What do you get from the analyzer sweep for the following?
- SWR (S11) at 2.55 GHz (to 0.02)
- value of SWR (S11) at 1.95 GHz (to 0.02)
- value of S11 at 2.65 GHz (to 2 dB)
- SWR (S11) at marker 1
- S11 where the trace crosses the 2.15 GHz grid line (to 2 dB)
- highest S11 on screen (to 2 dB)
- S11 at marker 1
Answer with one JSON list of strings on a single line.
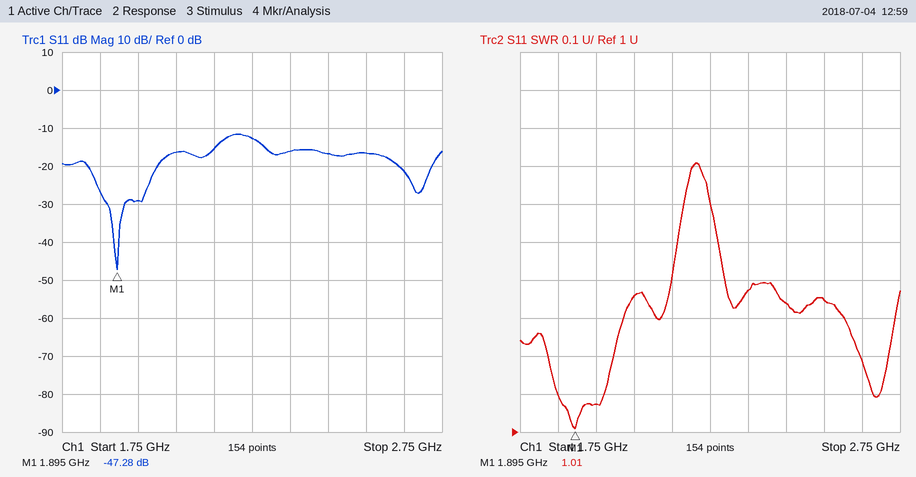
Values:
["1.34", "1.08", "-22 dB", "1.01", "-16 dB", "-12 dB", "-47.28 dB"]
